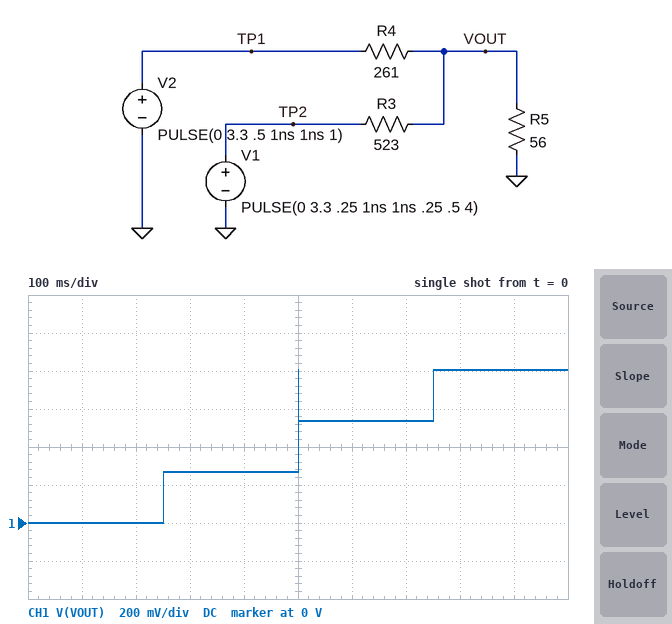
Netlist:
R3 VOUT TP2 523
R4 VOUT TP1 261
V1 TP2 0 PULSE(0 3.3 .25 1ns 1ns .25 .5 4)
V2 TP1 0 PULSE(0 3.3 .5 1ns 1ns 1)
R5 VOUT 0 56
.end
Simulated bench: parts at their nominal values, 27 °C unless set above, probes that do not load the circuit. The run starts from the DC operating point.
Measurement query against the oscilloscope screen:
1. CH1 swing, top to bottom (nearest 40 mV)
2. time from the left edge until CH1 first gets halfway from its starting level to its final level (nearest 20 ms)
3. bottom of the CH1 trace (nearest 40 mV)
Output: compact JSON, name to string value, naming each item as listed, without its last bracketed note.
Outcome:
{"CH1 swing, top to bottom": "800 mV", "time from the left edge until CH1 first gets halfway from its starting level to its final level": "500 ms", "bottom of the CH1 trace": "0 V"}
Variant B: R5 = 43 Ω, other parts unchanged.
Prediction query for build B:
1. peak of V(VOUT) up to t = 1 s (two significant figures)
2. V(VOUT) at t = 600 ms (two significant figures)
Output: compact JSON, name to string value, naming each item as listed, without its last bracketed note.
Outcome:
{"peak of V(VOUT) up to t = 1 s": "650 mV", "V(VOUT) at t = 600 ms": "440 mV"}
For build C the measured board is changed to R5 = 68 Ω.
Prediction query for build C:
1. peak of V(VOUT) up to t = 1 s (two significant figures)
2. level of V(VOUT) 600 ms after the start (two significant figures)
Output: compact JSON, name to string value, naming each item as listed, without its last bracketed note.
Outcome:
{"peak of V(VOUT) up to t = 1 s": "930 mV", "level of V(VOUT) 600 ms after the start": "620 mV"}
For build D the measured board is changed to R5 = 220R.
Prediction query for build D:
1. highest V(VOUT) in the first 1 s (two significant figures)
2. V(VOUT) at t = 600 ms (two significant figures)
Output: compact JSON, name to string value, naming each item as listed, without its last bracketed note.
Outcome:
{"highest V(VOUT) in the first 1 s": "1.8 V", "V(VOUT) at t = 600 ms": "1.2 V"}
